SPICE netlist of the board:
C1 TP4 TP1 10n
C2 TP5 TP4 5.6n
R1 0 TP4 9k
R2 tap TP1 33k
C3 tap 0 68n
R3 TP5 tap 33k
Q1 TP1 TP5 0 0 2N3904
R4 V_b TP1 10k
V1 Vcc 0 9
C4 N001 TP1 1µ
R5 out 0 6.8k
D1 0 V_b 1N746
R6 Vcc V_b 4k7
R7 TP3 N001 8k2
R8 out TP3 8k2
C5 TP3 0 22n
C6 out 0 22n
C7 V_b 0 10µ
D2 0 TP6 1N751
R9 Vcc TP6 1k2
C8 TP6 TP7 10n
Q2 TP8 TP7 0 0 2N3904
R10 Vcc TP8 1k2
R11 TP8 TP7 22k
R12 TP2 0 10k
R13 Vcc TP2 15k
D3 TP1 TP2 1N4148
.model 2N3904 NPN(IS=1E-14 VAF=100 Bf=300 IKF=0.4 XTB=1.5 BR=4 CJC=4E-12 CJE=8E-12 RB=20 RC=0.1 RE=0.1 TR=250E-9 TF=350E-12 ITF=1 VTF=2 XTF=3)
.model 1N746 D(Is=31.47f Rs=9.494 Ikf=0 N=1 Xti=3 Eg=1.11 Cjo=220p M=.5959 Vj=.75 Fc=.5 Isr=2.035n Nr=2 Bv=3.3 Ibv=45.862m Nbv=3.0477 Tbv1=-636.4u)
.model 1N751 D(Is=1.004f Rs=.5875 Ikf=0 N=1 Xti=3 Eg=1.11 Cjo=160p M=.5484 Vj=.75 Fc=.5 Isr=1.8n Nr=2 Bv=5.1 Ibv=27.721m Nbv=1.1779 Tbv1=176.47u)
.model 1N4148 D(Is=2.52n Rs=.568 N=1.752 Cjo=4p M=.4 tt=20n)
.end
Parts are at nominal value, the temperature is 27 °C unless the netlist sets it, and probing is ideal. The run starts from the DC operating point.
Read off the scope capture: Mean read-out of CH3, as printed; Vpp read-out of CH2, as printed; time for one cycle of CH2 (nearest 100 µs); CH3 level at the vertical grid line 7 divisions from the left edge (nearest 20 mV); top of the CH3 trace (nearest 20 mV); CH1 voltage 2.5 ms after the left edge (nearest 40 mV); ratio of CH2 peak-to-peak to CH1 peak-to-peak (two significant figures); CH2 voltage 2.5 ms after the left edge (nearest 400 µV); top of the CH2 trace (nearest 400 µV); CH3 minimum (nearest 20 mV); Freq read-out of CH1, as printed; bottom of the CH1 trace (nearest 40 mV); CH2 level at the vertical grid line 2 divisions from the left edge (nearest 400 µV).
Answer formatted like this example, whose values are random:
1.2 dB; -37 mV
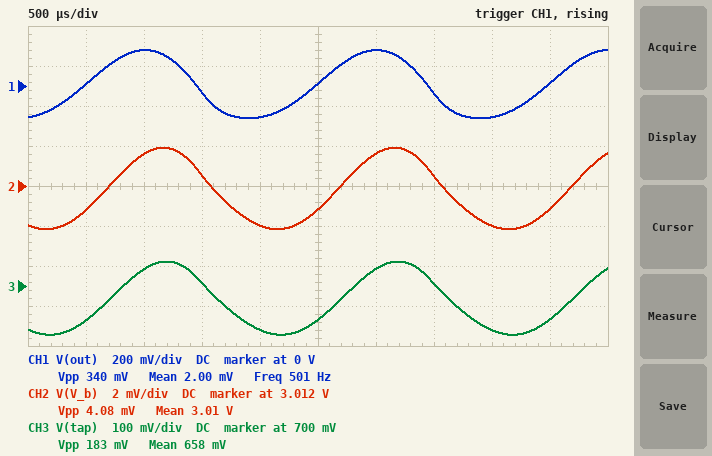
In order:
658 mV; 4.08 mV; 2.0 ms; 700 mV; 760 mV; 0 V; 0.012; 3.0108 V; 3.0140 V; 580 mV; 501 Hz; -160 mV; 3.0136 V
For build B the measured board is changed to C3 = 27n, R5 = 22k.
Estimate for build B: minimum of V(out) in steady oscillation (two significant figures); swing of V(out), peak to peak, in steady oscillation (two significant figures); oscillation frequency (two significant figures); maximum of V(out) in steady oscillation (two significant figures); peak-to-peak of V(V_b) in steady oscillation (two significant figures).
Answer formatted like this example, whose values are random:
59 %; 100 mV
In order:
-220 mV; 470 mV; 670 Hz; 250 mV; 3.1 mV
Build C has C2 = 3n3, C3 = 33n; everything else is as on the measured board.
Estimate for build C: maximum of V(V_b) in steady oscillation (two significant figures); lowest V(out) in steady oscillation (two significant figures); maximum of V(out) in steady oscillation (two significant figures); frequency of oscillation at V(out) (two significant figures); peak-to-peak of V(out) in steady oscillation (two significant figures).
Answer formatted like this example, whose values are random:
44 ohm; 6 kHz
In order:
3.0 V; -140 mV; 150 mV; 760 Hz; 290 mV
